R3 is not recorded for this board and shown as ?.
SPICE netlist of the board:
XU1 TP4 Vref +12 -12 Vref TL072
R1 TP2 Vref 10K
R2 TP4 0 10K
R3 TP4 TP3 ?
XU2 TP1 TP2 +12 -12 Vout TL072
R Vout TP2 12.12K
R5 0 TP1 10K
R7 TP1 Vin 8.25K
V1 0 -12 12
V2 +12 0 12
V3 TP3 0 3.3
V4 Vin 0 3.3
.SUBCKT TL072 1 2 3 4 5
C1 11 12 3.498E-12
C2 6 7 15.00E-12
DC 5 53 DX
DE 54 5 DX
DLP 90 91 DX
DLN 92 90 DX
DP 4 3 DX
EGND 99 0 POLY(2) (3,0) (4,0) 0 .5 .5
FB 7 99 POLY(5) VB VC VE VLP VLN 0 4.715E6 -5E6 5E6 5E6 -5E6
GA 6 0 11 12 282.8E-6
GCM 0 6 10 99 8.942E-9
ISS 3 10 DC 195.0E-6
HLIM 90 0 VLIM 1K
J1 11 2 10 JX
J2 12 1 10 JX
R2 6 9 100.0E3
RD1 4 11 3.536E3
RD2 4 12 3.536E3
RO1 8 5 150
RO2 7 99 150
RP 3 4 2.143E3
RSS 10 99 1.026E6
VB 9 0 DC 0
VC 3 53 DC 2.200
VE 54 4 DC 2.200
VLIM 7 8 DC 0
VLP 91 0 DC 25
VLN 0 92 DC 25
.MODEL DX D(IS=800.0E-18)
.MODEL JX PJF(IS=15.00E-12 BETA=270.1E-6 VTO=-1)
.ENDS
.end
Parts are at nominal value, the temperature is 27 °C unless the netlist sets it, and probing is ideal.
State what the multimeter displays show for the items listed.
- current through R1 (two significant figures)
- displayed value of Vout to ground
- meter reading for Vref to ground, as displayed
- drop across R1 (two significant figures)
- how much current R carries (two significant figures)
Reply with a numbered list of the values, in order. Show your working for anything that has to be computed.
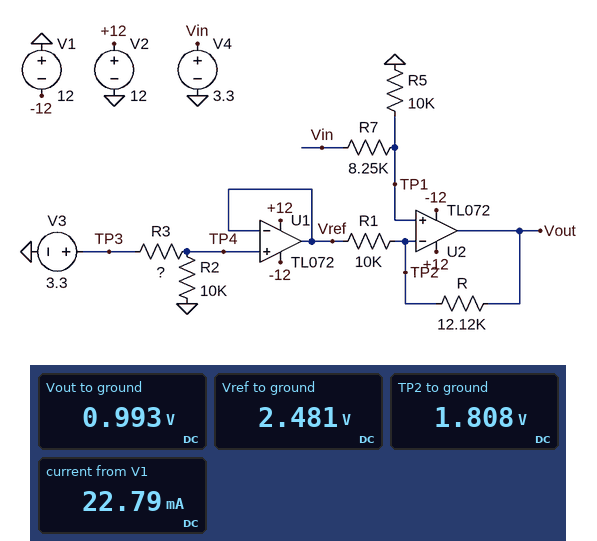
1. (2.481 V - 1.808 V) / 10 kΩ = 67 µA
2. 0.993 V
3. 2.481 V
4. 2.481 V - 1.808 V = 670 mV
5. (1.808 V - 993 mV) / 12.12 kΩ = 67 µA
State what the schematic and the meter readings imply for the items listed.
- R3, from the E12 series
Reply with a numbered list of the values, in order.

1. 3.3 kΩ
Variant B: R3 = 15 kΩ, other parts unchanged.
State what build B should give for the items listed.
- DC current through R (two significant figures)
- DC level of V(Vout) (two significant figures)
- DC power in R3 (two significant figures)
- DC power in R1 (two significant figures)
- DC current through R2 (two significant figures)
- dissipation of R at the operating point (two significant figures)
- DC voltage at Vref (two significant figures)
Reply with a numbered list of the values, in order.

1. 49 µA
2. 2.4 V
3. 260 µW
4. 24 µW
5. 130 µA
6. 29 µW
7. 1.3 V
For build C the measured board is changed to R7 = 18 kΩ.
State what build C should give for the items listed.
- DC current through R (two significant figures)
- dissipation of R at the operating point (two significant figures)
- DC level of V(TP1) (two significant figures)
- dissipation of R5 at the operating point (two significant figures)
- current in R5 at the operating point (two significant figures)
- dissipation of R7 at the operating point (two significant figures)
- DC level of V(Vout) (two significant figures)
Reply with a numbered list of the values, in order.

1. 130 µA
2. 210 µW
3. 1.2 V
4. 140 µW
5. 120 µA
6. 250 µW
7. -400 mV
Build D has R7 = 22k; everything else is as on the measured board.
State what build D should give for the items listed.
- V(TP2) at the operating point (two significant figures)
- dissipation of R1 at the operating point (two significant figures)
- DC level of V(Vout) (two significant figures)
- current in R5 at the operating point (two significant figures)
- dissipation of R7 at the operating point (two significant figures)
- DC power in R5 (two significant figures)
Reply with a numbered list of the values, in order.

1. 1.0 V
2. 210 µW
3. -730 mV
4. 100 µA
5. 230 µW
6. 110 µW
